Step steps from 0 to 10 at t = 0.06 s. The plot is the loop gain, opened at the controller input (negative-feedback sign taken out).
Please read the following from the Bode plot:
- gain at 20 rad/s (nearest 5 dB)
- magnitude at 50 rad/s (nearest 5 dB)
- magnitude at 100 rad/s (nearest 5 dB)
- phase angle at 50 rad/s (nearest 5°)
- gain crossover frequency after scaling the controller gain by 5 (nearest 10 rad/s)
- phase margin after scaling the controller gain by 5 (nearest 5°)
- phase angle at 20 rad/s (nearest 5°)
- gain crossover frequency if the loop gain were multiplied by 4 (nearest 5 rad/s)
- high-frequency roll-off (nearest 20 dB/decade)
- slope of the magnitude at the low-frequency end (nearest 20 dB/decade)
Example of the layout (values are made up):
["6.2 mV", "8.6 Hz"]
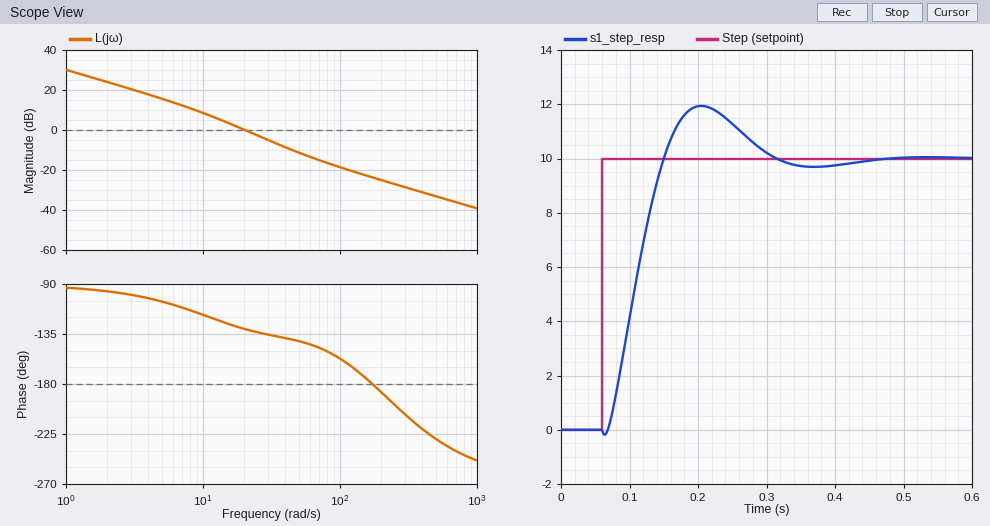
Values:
["0 dB", "-10 dB", "-20 dB", "-140°", "60 rad/s", "35°", "-130°", "55 rad/s", "-20 dB/decade", "-20 dB/decade"]
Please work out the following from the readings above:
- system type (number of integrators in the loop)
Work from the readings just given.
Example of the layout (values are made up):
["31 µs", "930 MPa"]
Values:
["1"]
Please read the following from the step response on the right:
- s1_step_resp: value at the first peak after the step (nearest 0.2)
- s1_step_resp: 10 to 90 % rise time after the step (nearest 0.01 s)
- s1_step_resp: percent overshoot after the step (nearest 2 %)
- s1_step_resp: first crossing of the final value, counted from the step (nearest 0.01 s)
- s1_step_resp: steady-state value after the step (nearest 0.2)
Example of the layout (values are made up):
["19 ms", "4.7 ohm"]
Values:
["12.0", "0.06 s", "20 %", "0.09 s", "10.0"]
